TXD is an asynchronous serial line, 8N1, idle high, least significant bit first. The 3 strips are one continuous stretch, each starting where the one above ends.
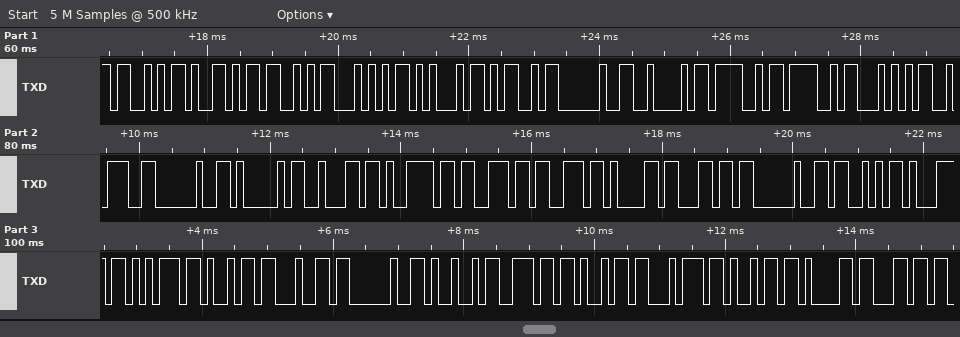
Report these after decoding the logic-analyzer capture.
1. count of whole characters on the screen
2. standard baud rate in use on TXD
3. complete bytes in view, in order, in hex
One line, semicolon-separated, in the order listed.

34; 9600 baud; 53 59 53 54 45 4D 20 42 4F 4F 54 3A 20 41 62 79 73 73 61 6C 20 53 71 75 69 64 20 49 6E 69 74 69 61 6C
